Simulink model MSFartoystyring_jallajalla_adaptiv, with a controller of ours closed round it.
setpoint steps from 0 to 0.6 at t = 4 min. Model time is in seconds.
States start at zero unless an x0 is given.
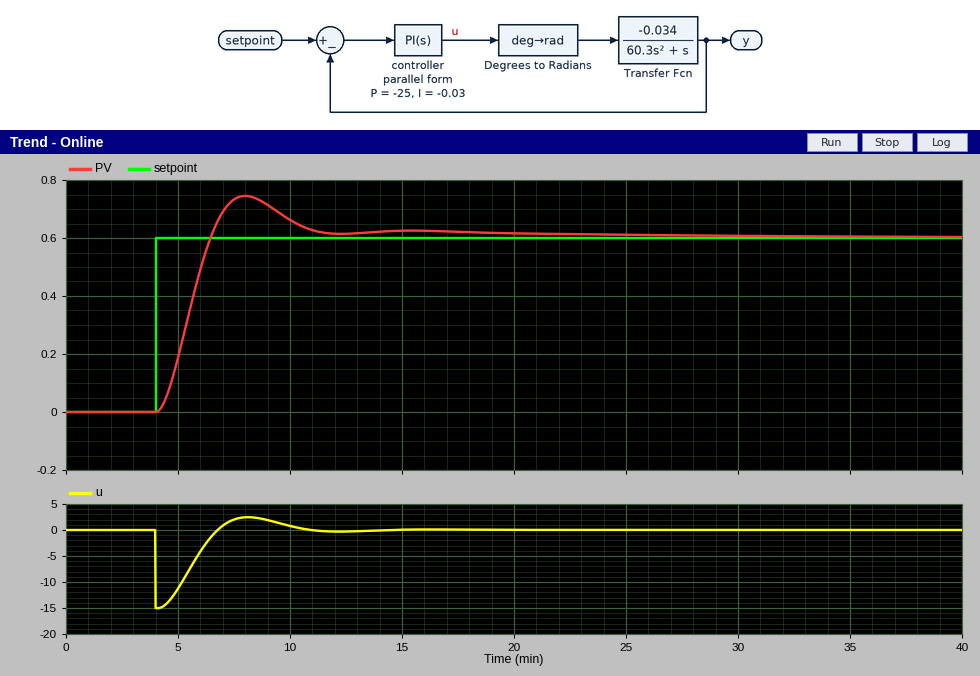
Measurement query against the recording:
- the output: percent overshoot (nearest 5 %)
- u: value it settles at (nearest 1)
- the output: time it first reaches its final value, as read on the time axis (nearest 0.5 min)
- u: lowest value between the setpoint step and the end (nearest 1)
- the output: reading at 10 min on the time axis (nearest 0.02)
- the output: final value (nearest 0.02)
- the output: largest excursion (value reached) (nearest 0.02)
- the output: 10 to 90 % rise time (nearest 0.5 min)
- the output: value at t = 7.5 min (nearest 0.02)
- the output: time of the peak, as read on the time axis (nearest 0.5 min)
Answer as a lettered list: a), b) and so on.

a) 25 %
b) 0
c) 6.5 min
d) -15
e) 0.66
f) 0.60
g) 0.74
h) 1.5 min
i) 0.74
j) 8.0 min
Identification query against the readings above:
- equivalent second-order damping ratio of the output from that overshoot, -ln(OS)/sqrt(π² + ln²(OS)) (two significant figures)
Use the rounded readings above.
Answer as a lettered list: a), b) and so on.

a) 0.40
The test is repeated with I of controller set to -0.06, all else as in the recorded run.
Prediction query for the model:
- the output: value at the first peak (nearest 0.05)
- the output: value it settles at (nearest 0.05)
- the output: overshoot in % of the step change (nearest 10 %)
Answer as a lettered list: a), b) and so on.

a) 0.80
b) 0.60
c) 30 %
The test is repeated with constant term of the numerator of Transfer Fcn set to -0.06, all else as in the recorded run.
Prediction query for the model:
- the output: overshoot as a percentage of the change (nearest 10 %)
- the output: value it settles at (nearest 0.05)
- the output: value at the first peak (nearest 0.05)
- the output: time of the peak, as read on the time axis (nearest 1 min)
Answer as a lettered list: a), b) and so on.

a) 30 %
b) 0.60
c) 0.80
d) 7 min
